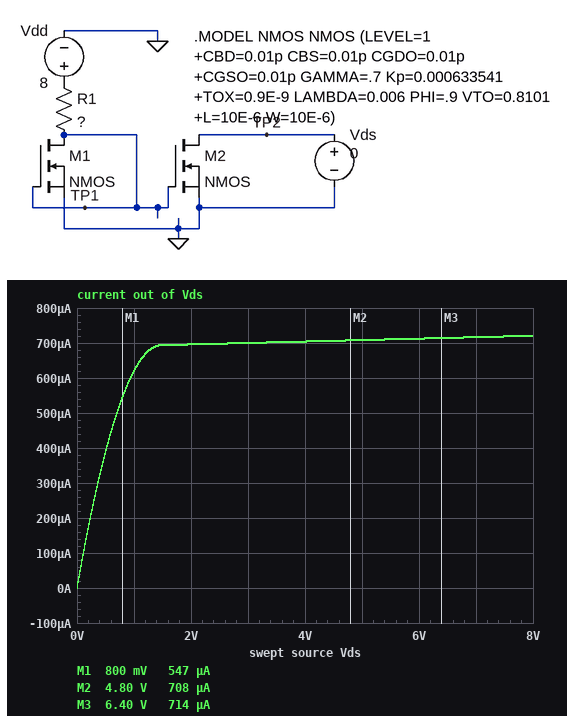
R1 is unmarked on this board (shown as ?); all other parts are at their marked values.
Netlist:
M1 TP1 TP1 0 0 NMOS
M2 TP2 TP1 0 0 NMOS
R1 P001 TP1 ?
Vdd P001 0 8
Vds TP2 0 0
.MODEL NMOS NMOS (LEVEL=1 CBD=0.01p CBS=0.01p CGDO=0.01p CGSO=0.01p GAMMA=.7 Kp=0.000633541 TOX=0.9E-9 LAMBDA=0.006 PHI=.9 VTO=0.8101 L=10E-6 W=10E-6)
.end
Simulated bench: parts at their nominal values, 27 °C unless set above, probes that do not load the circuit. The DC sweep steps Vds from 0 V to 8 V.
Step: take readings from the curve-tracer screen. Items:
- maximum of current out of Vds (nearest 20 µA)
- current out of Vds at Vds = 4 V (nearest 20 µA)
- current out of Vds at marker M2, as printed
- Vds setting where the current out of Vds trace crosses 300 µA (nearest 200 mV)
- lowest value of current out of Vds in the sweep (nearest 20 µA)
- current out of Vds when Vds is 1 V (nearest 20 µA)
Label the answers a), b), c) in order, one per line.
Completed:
a) 720 µA
b) 700 µA
c) 708 µA
d) 400 mV
e) 0 A
f) 620 µA
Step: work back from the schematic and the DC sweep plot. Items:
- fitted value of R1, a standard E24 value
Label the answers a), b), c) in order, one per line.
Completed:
a) 8.2 kΩ
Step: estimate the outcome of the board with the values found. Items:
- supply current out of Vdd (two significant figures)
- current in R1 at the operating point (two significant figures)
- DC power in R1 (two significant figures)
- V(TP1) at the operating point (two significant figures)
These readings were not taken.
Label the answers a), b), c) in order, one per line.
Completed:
a) 700 µA
b) 700 µA
c) 4.0 mW
d) 2.3 V
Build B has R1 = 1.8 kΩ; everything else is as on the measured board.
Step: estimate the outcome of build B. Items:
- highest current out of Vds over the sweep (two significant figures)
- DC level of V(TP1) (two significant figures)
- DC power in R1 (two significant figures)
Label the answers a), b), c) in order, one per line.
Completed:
a) 2.5 mA
b) 3.6 V
c) 11 mW
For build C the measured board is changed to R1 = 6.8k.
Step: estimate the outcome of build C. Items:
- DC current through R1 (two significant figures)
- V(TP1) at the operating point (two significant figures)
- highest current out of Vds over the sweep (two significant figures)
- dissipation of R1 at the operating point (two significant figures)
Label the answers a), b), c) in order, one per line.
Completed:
a) 820 µA
b) 2.4 V
c) 850 µA
d) 4.6 mW
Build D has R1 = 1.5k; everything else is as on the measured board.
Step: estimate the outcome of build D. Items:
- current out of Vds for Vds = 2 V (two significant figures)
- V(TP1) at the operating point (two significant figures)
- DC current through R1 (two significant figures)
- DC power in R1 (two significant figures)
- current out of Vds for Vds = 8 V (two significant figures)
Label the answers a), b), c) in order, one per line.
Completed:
a) 2.5 mA
b) 3.8 V
c) 2.8 mA
d) 12 mW
e) 2.9 mA
